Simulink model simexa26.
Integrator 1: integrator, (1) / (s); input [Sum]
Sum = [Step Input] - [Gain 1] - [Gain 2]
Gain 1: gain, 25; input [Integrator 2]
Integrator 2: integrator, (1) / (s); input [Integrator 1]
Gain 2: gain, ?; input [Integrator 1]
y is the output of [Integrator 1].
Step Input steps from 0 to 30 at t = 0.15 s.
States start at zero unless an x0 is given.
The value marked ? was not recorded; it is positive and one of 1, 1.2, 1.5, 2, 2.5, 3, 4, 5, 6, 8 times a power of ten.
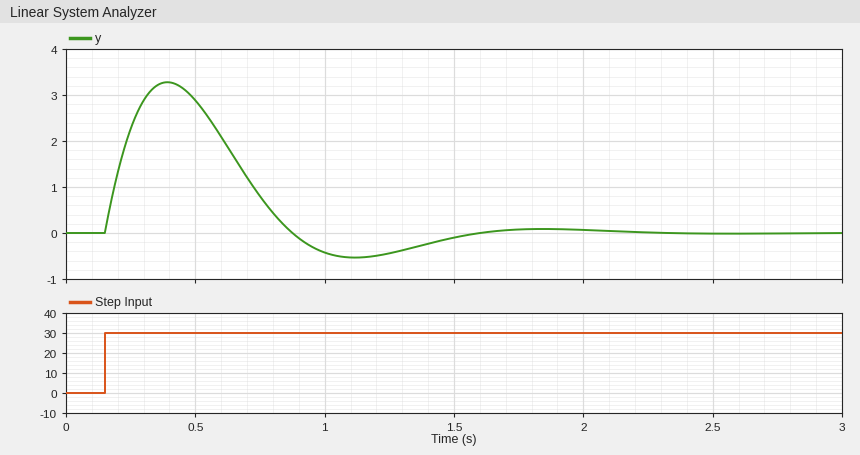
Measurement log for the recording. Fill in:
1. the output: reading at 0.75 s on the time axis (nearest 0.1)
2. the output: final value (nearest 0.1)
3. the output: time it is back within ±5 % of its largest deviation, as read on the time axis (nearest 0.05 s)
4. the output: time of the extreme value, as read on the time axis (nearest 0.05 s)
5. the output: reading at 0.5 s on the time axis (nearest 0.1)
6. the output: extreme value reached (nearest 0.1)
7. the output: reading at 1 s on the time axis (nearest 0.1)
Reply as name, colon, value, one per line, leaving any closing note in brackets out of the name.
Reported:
the output: reading at 0.75 s on the time axis: 0.8
the output: final value: 0.0
the output: time it is back within ±5 % of its largest deviation, as read on the time axis: 1.45 s
the output: time of the extreme value, as read on the time axis: 0.40 s
the output: reading at 0.5 s on the time axis: 2.9
the output: extreme value reached: 3.3
the output: reading at 1 s on the time axis: -0.4
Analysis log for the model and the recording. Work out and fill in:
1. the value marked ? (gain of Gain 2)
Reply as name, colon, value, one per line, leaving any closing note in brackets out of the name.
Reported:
the value marked ?: 5
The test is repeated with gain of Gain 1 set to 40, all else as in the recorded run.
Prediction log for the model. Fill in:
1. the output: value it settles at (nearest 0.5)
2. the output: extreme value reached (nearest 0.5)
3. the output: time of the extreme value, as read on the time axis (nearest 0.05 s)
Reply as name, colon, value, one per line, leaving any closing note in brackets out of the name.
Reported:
the output: value it settles at: 0.0
the output: extreme value reached: 3.0
the output: time of the extreme value, as read on the time axis: 0.35 s
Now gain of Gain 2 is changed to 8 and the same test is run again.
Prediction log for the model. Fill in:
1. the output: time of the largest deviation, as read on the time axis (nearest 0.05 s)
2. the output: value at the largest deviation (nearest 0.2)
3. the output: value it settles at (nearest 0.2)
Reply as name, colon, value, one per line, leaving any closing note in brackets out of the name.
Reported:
the output: time of the largest deviation, as read on the time axis: 0.35 s
the output: value at the largest deviation: 2.6
the output: value it settles at: 0.0
